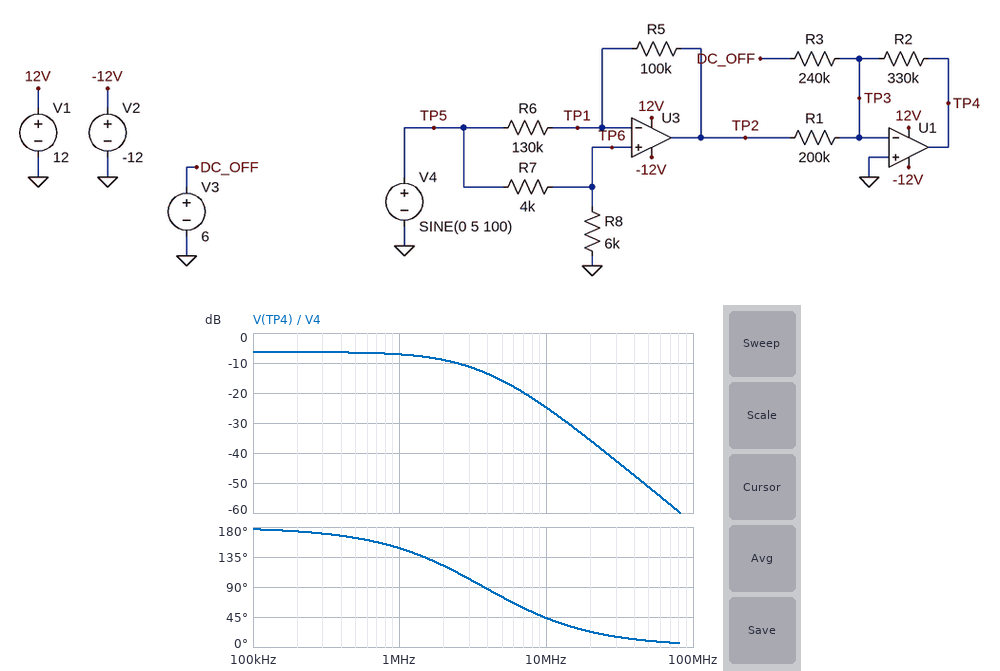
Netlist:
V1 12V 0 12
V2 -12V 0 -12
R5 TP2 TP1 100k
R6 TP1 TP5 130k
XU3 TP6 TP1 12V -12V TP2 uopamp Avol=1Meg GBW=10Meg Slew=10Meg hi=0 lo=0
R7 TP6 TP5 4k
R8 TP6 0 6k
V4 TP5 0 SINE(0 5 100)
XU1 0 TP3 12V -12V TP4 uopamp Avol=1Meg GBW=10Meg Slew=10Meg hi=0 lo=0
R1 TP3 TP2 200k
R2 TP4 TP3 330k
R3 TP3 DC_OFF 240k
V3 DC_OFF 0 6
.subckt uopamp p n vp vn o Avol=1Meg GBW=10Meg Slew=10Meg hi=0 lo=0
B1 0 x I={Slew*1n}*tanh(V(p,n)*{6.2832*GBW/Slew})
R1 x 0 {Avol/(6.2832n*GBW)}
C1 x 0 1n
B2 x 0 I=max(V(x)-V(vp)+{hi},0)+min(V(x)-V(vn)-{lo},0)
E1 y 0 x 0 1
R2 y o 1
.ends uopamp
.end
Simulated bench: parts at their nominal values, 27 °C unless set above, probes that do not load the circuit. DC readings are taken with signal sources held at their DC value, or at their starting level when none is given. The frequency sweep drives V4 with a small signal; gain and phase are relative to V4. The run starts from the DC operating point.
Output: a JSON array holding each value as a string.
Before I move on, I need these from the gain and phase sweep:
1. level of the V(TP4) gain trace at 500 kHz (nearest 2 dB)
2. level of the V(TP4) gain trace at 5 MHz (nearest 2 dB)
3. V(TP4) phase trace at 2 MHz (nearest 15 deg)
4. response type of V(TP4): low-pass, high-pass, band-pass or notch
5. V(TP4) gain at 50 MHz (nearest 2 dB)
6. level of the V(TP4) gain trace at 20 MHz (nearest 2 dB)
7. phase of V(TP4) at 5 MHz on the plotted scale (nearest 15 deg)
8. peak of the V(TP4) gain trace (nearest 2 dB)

["-6 dB", "-16 dB", "120 deg", "low-pass", "-52 dB", "-36 dB", "75 deg", "-6 dB"]
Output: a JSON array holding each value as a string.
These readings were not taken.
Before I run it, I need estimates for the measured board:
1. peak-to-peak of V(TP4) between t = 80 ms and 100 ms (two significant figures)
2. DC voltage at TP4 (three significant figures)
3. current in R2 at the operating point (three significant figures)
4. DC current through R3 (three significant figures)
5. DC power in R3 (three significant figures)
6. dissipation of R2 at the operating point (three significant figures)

["4.8 V", "-8.25 V", "25.0 µA", "25.0 µA", "150 µW", "206 µW"]
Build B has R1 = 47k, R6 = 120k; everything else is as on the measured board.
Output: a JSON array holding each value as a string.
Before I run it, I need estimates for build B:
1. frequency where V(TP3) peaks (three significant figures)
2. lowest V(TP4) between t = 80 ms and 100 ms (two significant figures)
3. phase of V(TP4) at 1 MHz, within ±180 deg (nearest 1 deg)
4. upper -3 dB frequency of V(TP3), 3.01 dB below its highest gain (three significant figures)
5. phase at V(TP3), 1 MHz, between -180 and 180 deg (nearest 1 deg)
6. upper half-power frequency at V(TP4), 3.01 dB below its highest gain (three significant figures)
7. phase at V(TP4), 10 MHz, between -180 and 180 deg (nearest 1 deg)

["2.41 MHz", "-12 V", "126 deg", "7.31 MHz", "36 deg", "1.03 MHz", "35 deg"]
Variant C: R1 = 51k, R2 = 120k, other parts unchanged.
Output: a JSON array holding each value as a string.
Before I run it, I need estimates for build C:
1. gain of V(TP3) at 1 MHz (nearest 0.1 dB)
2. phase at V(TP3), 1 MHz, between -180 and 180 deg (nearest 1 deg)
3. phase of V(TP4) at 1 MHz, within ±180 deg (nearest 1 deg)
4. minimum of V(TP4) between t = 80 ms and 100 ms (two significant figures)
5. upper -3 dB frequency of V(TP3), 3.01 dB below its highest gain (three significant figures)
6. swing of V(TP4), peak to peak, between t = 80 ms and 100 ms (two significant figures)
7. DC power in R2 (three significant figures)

["-24.0 dB", "59 deg", "149 deg", "-6.4 V", "9.75 MHz", "6.9 V", "75.0 µW"]
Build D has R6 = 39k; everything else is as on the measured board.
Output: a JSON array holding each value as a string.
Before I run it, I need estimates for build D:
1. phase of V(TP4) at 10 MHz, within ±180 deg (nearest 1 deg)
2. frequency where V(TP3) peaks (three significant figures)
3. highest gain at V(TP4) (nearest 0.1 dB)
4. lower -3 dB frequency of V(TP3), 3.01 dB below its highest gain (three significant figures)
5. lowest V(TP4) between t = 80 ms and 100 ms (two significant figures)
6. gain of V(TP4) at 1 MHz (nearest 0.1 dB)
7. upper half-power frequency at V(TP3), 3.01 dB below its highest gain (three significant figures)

["-150 deg", "2.64 MHz", "-3.1 dB", "1.09 MHz", "-12 V", "-4.2 dB", "6.38 MHz"]
